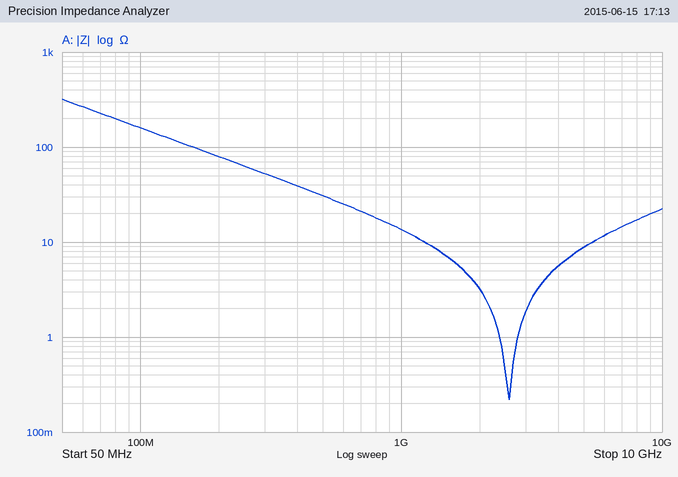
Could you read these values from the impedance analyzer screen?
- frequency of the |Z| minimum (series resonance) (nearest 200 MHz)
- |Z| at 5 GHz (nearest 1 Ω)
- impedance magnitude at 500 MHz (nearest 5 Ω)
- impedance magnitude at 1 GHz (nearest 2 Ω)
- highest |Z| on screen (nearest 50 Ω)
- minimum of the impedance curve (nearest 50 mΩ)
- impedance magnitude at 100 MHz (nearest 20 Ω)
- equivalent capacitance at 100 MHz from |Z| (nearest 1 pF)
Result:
2.6 GHz
9 Ω
30 Ω
14 Ω
300 Ω
200 mΩ
160 Ω
10 pF
